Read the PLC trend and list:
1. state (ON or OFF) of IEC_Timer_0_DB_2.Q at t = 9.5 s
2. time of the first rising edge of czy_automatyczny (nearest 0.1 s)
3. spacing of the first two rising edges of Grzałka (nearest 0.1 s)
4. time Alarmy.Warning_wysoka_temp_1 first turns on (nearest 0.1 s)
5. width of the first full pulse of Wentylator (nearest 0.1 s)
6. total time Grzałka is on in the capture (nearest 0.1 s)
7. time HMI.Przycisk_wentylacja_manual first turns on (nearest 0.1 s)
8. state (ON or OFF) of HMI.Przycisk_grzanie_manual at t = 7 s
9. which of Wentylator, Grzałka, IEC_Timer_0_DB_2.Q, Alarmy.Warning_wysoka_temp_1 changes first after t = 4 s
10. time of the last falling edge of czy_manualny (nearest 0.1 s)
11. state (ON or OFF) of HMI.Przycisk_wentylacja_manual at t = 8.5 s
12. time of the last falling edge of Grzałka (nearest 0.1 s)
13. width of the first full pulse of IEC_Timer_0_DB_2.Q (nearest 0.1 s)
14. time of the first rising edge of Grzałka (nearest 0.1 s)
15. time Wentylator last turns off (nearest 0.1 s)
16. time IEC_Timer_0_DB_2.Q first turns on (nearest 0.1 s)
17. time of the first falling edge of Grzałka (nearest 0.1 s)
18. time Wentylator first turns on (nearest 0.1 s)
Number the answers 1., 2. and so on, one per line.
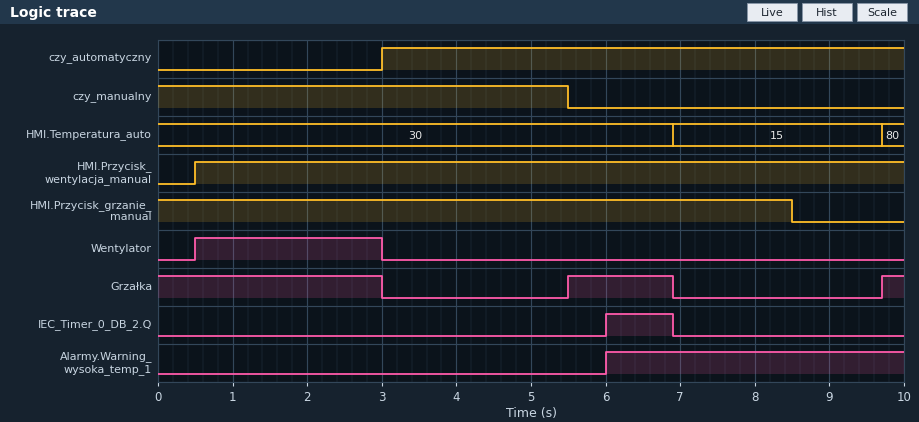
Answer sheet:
1. OFF
2. 3.0 s
3. 4.2 s
4. 6.0 s
5. 2.5 s
6. 4.7 s
7. 0.5 s
8. ON
9. Grzałka
10. 5.5 s
11. ON
12. 6.9 s
13. 0.9 s
14. 5.5 s
15. 3.0 s
16. 6.0 s
17. 3.0 s
18. 0.5 s
